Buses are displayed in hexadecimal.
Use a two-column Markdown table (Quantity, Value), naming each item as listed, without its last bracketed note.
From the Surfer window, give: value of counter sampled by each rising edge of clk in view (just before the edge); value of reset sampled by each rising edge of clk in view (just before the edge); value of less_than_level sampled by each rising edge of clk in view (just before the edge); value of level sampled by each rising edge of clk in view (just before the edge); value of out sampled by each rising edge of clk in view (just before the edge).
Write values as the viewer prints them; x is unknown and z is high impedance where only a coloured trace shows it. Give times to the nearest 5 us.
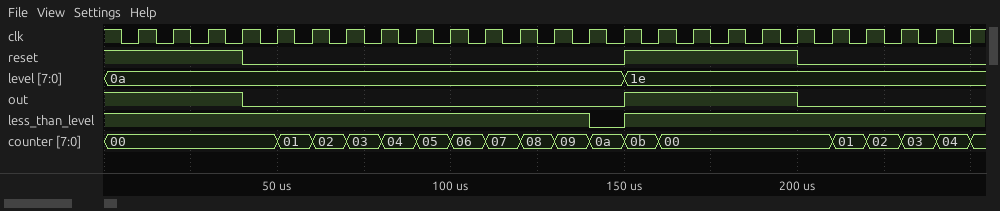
| Quantity | Value |
|---|---|
| value of counter sampled by each rising edge of clk in view | 00, 00, 00, 00, 00, 01, 02, 03, 04, 05, 06, 07, 08, 09, 0a, 0b, 00, 00, 00, 00, 00, 01, 02, 03, 04 |
| value of reset sampled by each rising edge of clk in view | 1 1 1 1 0 0 0 0 0 0 0 0 0 0 0 1 1 1 1 1 0 0 0 0 0 |
| value of less_than_level sampled by each rising edge of clk in view | 1 1 1 1 1 1 1 1 1 1 1 1 1 1 0 1 1 1 1 1 1 1 1 1 1 |
| value of level sampled by each rising edge of clk in view | 0a, 0a, 0a, 0a, 0a, 0a, 0a, 0a, 0a, 0a, 0a, 0a, 0a, 0a, 0a, 1e, 1e, 1e, 1e, 1e, 1e, 1e, 1e, 1e, 1e |
| value of out sampled by each rising edge of clk in view | 1 1 1 1 0 0 0 0 0 0 0 0 0 0 0 1 1 1 1 1 0 0 0 0 0 |
